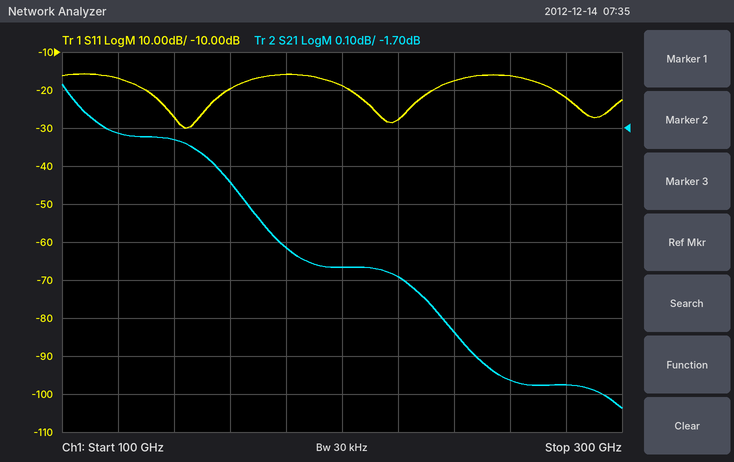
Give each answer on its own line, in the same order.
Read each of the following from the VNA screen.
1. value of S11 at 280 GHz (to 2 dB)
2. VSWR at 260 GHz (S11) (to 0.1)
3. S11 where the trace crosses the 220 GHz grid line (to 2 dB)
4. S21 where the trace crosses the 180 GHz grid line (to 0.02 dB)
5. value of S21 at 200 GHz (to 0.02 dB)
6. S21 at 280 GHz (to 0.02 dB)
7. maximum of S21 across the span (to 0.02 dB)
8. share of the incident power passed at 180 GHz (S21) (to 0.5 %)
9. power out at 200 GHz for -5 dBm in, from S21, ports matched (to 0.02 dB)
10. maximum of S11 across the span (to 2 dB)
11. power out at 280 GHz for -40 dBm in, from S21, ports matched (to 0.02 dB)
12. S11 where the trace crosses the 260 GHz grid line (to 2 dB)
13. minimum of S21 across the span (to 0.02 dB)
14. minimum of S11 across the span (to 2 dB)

-22 dB
1.4
-28 dB
-2.02 dB
-2.06 dB
-2.38 dB
-1.58 dB
63.0 %
-7.06 dBm
-16 dB
-42.38 dBm
-16 dB
-2.44 dB
-30 dB
